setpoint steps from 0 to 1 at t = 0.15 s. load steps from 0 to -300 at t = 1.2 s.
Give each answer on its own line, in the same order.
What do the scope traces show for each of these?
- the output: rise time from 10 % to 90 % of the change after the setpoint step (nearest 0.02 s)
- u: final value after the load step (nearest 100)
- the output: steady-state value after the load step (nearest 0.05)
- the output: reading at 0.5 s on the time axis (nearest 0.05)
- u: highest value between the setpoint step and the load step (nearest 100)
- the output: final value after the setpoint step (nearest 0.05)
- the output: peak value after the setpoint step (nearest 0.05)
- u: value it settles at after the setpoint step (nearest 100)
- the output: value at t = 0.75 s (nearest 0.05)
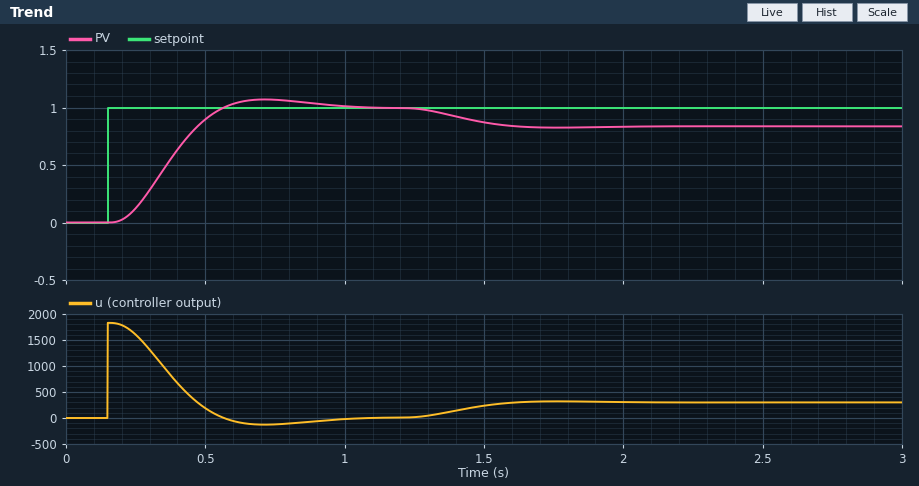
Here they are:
0.26 s
300
0.85
0.90
1800
1.00
1.05
0
1.05
